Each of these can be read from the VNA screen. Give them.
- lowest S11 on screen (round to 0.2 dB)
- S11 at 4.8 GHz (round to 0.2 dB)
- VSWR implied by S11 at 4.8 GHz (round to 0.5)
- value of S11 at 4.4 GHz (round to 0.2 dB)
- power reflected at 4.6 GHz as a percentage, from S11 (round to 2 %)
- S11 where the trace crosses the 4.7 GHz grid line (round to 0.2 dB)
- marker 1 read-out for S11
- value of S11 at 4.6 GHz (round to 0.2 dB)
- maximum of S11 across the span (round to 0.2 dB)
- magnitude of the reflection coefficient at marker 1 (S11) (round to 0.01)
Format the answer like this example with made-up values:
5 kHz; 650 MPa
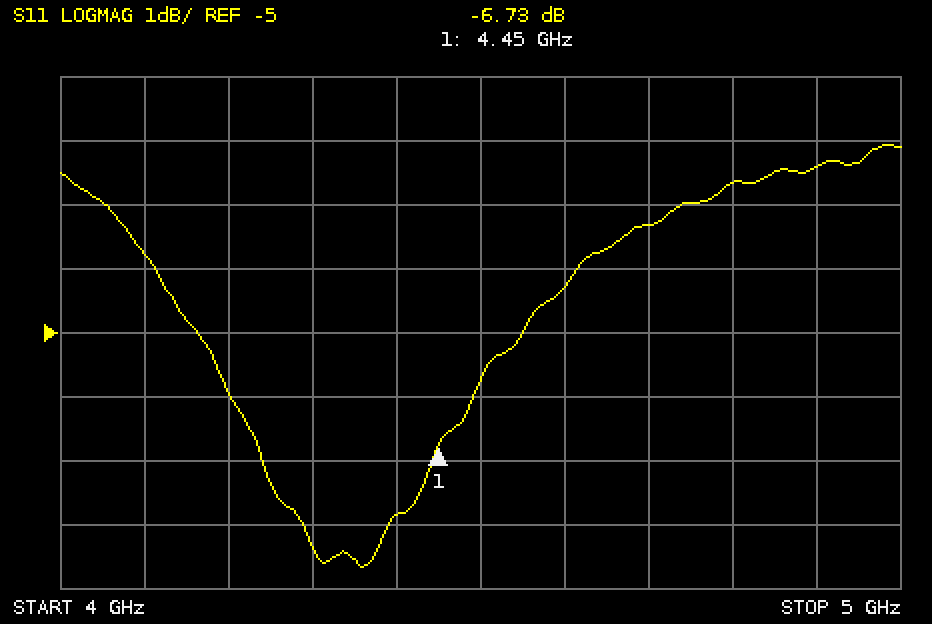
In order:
-8.6 dB; -2.6 dB; 6.5; -7.8 dB; 38 %; -3.4 dB; -6.73 dB; -4.2 dB; -2.0 dB; 0.46
